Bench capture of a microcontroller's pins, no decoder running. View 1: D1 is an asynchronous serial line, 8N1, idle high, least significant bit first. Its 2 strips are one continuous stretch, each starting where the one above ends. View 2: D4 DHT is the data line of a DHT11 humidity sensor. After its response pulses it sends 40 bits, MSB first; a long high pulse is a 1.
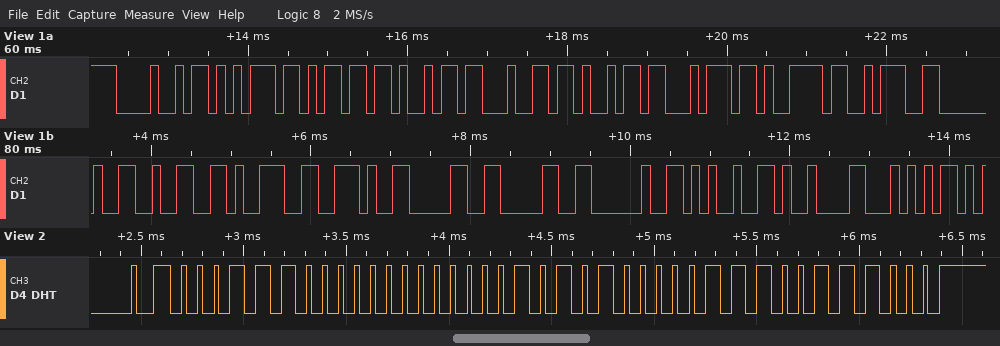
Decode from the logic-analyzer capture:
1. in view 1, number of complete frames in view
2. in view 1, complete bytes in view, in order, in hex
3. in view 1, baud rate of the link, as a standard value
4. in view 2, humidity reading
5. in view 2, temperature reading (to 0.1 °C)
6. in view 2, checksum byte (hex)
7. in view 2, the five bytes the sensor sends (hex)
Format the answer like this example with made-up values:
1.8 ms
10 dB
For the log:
19
48 75 6D 69 64 69 74 79 3A 20 32 39 2E 30 30 20 25 09 54
9600 baud
28 %
21.7 °C
0x38
1C 00 15 07 38
